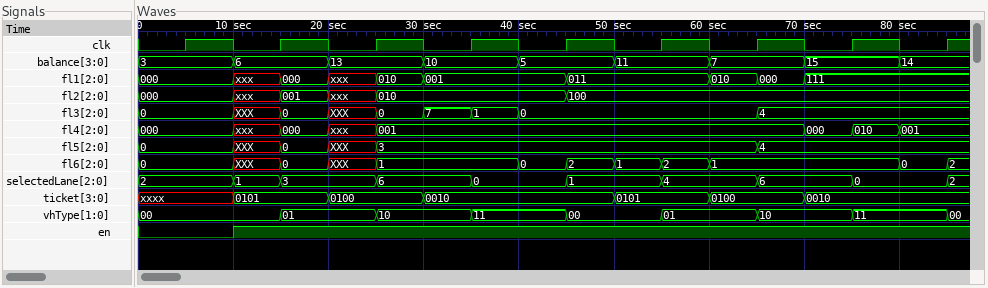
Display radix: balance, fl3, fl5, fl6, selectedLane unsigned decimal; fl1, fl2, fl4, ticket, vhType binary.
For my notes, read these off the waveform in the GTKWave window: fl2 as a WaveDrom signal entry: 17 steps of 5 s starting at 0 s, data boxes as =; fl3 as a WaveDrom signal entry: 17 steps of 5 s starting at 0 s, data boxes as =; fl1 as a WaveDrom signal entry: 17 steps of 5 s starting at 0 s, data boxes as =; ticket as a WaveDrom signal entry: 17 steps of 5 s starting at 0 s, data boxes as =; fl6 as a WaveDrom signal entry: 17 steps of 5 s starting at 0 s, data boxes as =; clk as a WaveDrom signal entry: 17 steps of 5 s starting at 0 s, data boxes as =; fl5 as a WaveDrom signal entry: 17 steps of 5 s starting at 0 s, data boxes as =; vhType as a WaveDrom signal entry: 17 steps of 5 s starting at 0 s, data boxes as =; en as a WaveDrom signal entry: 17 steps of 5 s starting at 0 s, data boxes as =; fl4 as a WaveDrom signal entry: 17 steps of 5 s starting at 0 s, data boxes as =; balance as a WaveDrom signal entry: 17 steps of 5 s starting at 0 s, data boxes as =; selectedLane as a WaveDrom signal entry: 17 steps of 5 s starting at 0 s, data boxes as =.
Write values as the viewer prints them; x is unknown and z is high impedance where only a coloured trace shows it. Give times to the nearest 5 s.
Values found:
{name: 'fl2', wave: '=.x=x=...=.......', data: '000 001 010 100'}
{name: 'fl3', wave: '=.x=x====....=...', data: '0 0 0 7 1 0 4'}
{name: 'fl1', wave: '=.x=x==..=..===..', data: '000 000 010 001 011 010 000 111'}
{name: 'ticket', wave: 'x.=.=.=...=.=.=..', data: '0101 0100 0010 0101 0100 0010'}
{name: 'fl6', wave: '=.x=x=..=====...=', data: '0 0 1 0 2 1 2 1 0'}
{name: 'clk', wave: '01010101010101010'}
{name: 'fl5', wave: '=.x=x=.......=...', data: '0 0 3 4'}
{name: 'vhType', wave: '=..=.=.=.=.=.=.=.', data: '00 01 10 11 00 01 10 11'}
{name: 'en', wave: '0.1..............'}
{name: 'fl4', wave: '=.x=x=........===', data: '000 000 001 000 010 001'}
{name: 'balance', wave: '=.=.=.=.=.=.=.=.=', data: '3 6 13 10 5 11 7 15 14'}
{name: 'selectedLane', wave: '=.==.=.=.=.=.=.=.', data: '2 1 3 6 0 1 4 6 0'}
